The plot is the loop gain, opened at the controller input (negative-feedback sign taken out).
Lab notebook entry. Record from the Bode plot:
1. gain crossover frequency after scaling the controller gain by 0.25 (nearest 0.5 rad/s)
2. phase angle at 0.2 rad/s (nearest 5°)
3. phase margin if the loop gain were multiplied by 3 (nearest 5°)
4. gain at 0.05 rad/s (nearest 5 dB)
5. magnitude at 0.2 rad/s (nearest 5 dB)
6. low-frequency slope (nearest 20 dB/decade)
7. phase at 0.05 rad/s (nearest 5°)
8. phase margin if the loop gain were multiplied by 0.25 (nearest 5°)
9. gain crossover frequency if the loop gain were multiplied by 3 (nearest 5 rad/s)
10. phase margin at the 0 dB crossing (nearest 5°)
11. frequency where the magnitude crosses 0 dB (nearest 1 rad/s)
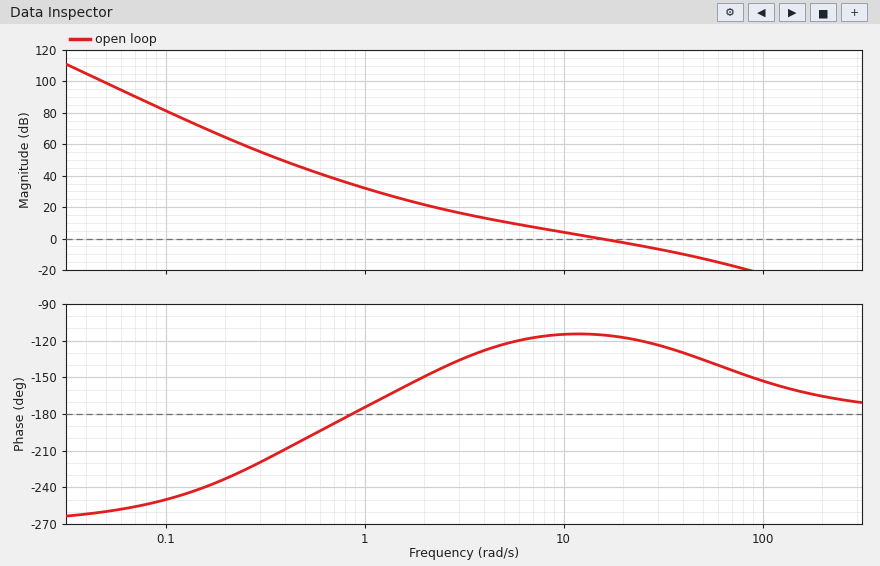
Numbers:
4.5 rad/s
-235°
50°
100 dB
65 dB
-60 dB/decade
-260°
55°
40 rad/s
65°
15 rad/s
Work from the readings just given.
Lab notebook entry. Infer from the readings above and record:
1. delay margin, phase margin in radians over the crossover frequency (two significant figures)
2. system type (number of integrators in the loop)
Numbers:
0.076 s
3
